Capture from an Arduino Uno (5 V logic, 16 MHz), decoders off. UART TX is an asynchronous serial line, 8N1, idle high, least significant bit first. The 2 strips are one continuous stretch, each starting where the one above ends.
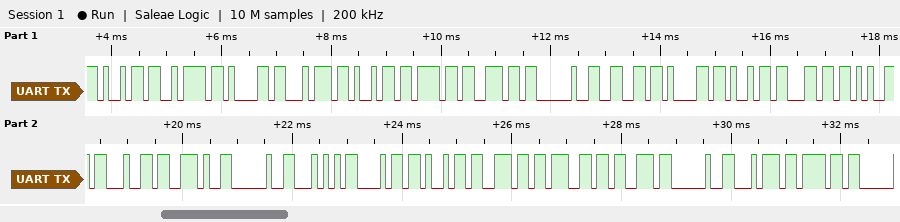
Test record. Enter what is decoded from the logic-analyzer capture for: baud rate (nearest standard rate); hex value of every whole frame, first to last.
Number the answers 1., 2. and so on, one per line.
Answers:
1. 9600 baud
2. 69 7A 61 74 69 6F 6E 20 66 61 69 6C 65 64 2E 20 54 68 69 6E 67 73 20 74 6F
